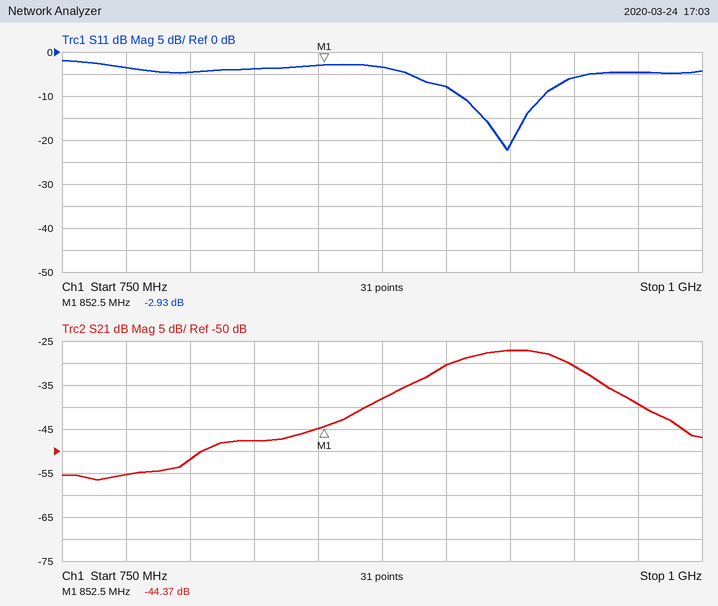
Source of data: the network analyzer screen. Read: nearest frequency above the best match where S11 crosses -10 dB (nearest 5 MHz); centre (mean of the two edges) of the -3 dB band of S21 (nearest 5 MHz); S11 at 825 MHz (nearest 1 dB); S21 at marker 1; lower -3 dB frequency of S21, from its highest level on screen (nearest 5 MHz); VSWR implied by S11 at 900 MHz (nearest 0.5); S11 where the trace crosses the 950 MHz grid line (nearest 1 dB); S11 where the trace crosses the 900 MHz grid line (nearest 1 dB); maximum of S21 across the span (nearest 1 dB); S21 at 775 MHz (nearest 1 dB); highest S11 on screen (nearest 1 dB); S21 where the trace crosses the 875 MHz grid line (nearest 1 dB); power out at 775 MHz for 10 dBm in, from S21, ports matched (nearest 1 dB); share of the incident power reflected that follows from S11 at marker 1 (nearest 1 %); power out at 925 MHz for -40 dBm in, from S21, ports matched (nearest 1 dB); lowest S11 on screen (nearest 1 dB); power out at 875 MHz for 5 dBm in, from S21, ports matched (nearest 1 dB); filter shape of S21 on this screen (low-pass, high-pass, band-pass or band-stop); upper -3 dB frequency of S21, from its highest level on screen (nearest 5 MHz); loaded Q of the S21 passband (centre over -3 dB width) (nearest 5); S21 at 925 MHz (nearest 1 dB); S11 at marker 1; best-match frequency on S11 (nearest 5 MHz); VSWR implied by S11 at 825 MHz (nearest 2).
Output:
940 MHz
925 MHz
-4 dB
-44.37 dB
900 MHz
2.5
-6 dB
-8 dB
-27 dB
-55 dB
-2 dB
-38 dB
-45 dBm
51 %
-67 dBm
-22 dB
-33 dBm
band-pass
950 MHz
20
-27 dB
-2.93 dB
925 MHz
4
